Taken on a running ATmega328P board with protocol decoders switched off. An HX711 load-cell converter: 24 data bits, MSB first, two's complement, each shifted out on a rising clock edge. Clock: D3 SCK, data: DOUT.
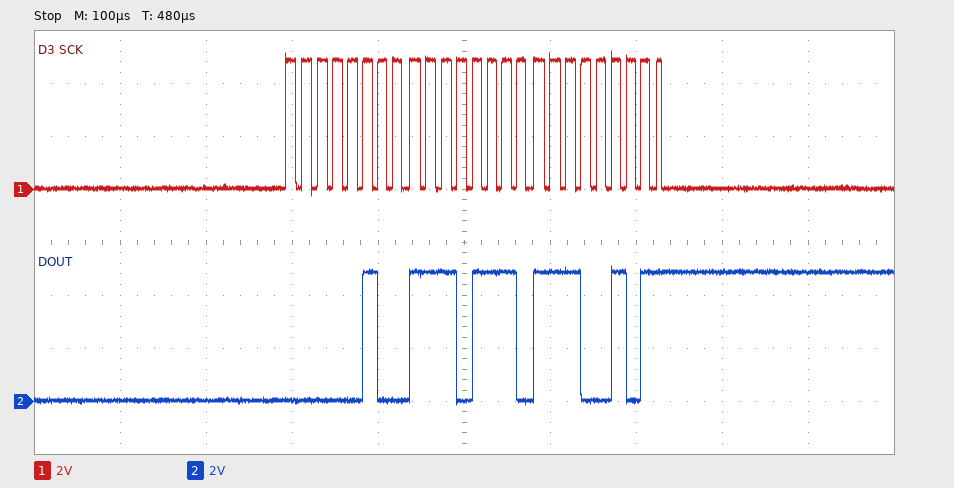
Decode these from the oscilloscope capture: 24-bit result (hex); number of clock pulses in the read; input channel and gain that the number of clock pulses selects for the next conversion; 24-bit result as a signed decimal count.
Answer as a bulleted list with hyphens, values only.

- 0x04EEE5
- 25
- channel A, gain 128
- 323301
